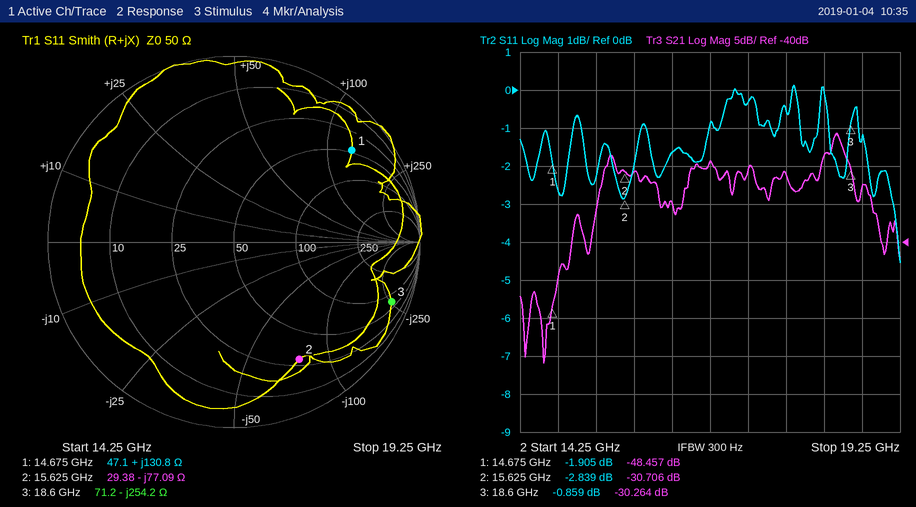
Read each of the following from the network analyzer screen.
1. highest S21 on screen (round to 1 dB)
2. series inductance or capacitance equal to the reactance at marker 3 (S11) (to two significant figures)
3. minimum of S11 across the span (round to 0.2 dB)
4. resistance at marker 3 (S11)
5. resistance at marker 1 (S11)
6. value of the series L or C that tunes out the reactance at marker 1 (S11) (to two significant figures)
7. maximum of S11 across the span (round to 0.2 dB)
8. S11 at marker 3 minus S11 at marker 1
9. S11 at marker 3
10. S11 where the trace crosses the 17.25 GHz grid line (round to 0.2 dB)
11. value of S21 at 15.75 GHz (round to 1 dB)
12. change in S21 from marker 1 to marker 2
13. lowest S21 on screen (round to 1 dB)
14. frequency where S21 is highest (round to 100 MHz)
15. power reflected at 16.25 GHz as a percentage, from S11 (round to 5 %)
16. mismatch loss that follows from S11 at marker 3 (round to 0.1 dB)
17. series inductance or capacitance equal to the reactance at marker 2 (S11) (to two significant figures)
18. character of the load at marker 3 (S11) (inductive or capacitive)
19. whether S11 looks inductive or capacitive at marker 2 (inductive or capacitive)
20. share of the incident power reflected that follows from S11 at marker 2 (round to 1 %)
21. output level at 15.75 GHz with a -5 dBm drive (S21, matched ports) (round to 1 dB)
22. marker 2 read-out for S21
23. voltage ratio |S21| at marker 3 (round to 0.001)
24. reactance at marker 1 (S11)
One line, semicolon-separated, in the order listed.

-26 dB; 34 fF; -4.6 dB; 71.2 Ω; 47.1 Ω; 83 fF; 0.2 dB; 1.046 dB; -0.859 dB; -0.4 dB; -31 dB; 17.751 dB; -56 dB; 18.4 GHz; 70 %; 7.5 dB; 130 fF; capacitive; capacitive; 52 %; -36 dBm; -30.706 dB; 0.031; +130.8 Ω
